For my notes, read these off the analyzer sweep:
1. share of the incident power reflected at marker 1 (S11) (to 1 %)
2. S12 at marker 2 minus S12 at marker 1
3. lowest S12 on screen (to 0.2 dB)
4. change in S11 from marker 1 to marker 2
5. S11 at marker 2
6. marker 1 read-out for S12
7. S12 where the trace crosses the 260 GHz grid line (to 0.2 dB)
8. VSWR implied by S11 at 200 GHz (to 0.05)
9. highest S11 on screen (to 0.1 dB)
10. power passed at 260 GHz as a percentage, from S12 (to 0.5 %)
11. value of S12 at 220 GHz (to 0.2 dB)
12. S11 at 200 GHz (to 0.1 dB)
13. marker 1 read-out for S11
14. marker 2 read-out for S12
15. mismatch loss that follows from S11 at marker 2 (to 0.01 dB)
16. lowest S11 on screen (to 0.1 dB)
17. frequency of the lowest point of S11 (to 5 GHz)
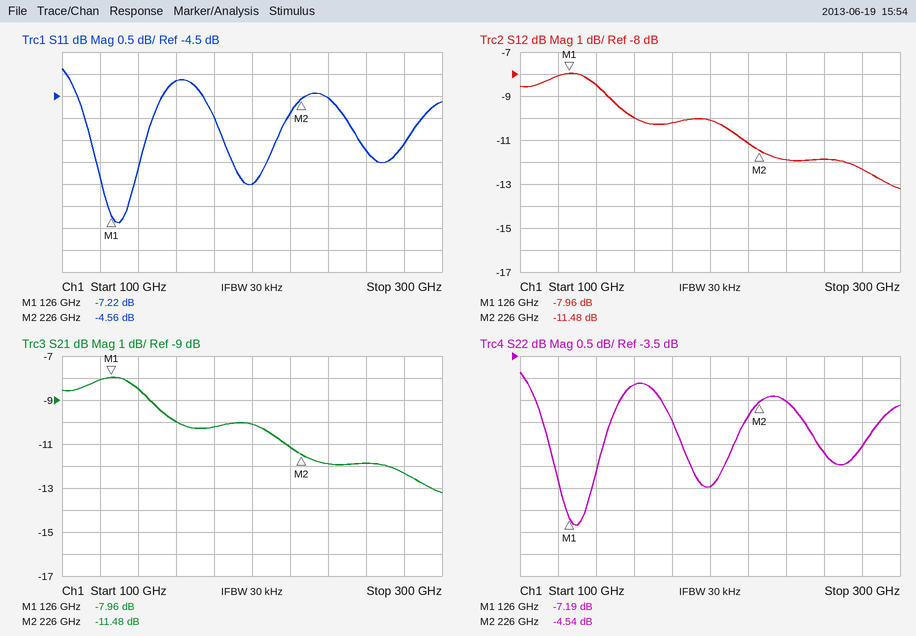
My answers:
19 %
-3.52 dB
-13.2 dB
2.66 dB
-4.56 dB
-7.96 dB
-11.8 dB
2.80
-3.9 dB
6.5 %
-11.2 dB
-6.5 dB
-7.22 dB
-11.48 dB
1.87 dB
-7.4 dB
130 GHz
